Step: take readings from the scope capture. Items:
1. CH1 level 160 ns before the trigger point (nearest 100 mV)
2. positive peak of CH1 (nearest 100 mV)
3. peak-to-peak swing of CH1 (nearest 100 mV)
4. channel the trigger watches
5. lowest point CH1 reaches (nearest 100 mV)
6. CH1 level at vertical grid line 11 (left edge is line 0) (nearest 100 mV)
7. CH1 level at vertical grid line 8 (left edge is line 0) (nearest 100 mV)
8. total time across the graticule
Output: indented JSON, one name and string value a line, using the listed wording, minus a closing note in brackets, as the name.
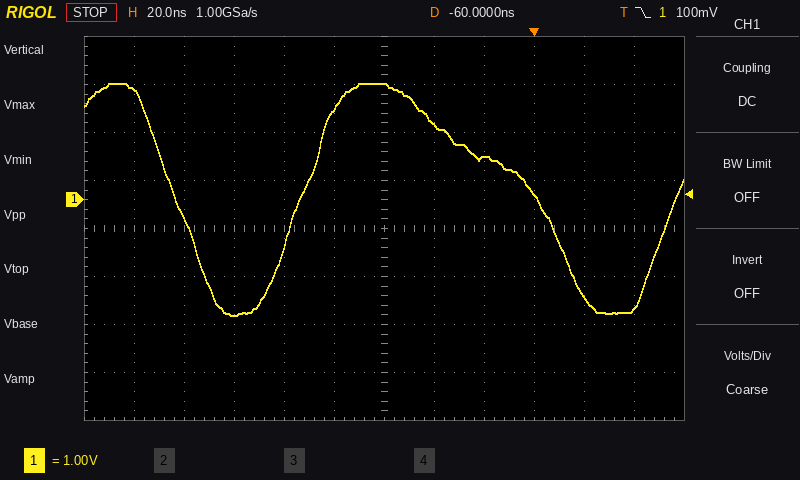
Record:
{
  "CH1 level 160 ns before the trigger point": "2.3 V",
  "positive peak of CH1": "2.4 V",
  "peak-to-peak swing of CH1": "4.8 V",
  "channel the trigger watches": "CH1",
  "lowest point CH1 reaches": "-2.4 V",
  "CH1 level at vertical grid line 11 (left edge is line 0)": "-2.3 V",
  "CH1 level at vertical grid line 8 (left edge is line 0)": "900 mV",
  "total time across the graticule": "240 ns"
}
